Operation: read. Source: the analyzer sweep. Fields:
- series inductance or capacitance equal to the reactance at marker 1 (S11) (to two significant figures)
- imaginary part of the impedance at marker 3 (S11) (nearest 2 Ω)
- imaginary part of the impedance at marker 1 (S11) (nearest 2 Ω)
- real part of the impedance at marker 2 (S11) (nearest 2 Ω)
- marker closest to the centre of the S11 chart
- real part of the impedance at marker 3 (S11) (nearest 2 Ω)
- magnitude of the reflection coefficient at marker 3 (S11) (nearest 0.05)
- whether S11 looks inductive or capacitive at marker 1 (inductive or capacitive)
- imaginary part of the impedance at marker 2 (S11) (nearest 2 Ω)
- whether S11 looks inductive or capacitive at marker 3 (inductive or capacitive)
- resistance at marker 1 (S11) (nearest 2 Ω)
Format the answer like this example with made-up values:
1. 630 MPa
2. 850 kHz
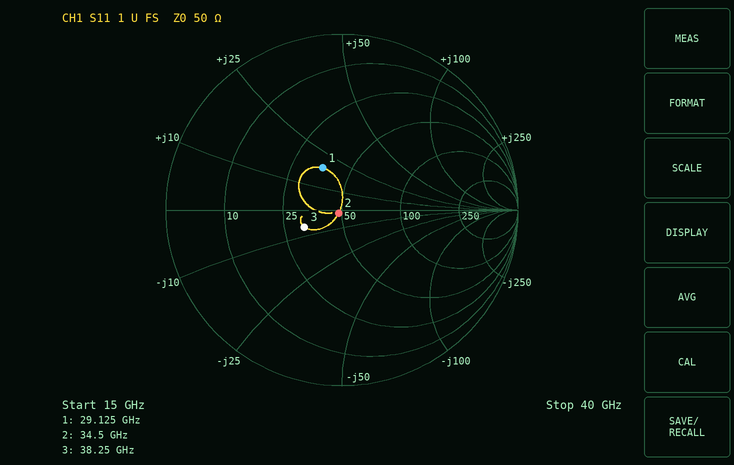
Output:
1. 100 pH
2. -6 Ω
3. +18 Ω
4. 48 Ω
5. marker 2
6. 32 Ω
7. 0.25
8. inductive
9. -2 Ω
10. capacitive
11. 36 Ω
